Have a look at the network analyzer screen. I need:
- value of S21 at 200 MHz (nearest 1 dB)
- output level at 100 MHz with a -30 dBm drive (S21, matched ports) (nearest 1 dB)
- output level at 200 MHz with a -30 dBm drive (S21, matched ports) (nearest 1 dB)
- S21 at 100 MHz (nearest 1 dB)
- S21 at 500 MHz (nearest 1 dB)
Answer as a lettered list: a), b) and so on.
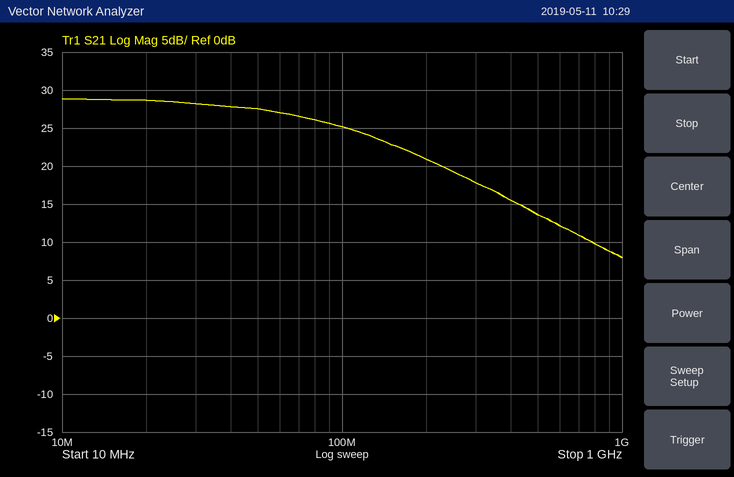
a) 21 dB
b) -5 dBm
c) -9 dBm
d) 25 dB
e) 14 dB
